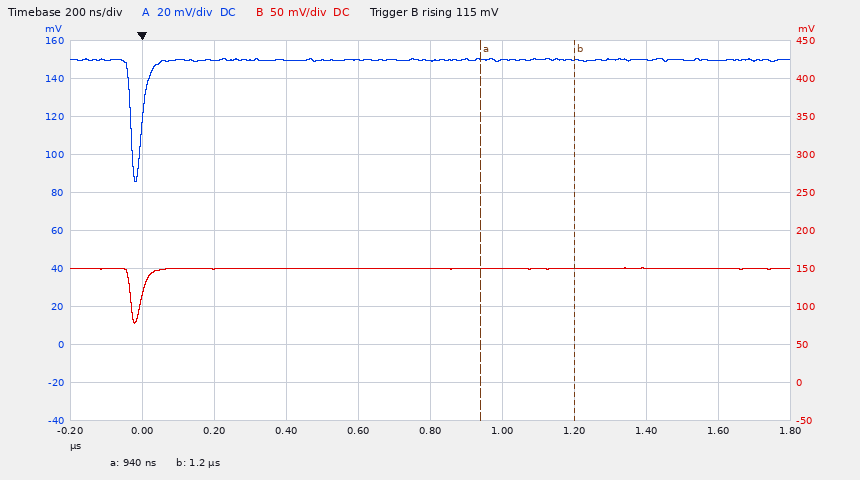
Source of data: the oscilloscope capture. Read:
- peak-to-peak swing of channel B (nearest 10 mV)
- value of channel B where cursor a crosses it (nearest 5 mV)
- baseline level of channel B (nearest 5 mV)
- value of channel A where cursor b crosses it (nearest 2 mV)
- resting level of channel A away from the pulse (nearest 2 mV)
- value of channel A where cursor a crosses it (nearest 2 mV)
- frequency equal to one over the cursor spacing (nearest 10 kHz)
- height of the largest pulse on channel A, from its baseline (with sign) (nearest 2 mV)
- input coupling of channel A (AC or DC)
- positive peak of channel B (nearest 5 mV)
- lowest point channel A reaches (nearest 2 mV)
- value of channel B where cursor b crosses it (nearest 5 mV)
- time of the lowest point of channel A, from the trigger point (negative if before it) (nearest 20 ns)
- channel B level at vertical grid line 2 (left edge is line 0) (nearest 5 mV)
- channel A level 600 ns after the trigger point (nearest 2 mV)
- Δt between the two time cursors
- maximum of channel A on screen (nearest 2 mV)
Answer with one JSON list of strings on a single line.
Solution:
["70 mV", "150 mV", "150 mV", "150 mV", "150 mV", "150 mV", "3.85 MHz", "-64 mV", "DC", "150 mV", "86 mV", "150 mV", "-20 ns", "150 mV", "150 mV", "260 ns", "150 mV"]
